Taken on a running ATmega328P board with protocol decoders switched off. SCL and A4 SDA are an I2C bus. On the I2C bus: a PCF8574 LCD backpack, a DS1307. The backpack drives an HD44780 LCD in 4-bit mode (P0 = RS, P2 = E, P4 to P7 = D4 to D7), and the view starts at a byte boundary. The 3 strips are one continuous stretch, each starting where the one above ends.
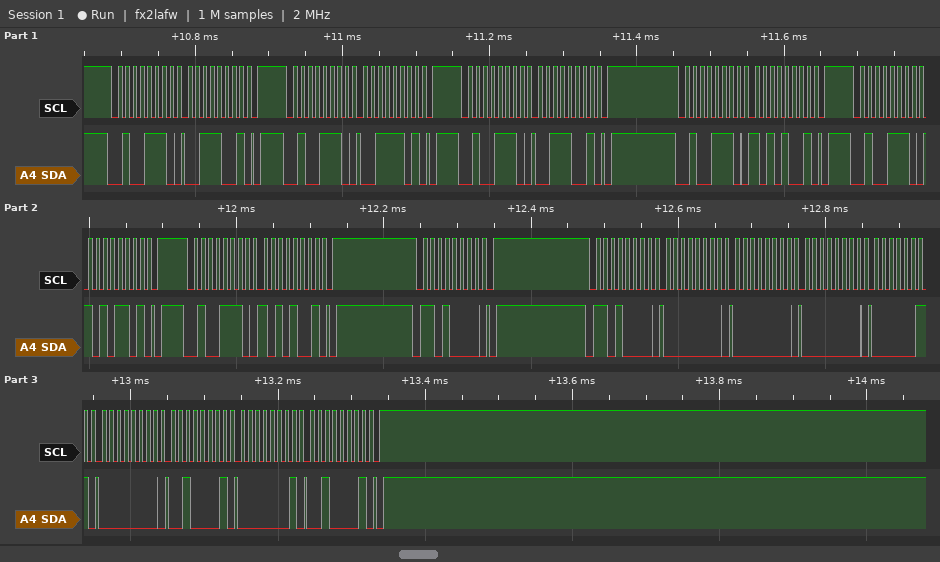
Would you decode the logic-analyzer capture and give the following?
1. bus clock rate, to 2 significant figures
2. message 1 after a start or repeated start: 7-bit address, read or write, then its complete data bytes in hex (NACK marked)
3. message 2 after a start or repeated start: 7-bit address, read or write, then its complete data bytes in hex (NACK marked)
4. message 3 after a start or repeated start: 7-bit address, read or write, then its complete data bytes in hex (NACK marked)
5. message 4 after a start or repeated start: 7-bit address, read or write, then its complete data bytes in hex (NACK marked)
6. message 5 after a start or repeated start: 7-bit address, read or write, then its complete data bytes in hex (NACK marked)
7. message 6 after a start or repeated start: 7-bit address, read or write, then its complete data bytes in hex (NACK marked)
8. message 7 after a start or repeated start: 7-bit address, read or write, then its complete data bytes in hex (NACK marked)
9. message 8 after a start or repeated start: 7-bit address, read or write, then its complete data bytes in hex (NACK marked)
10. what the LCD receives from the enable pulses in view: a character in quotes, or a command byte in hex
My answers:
100 kHz
0x27 write: 39
0x27 write: 3D
0x27 write: 39
0x27 write: A9
0x27 write: AD
0x27 write: A9
0x68 write
0x68 write: 00 00 00 03 00 21 01 21
':'
